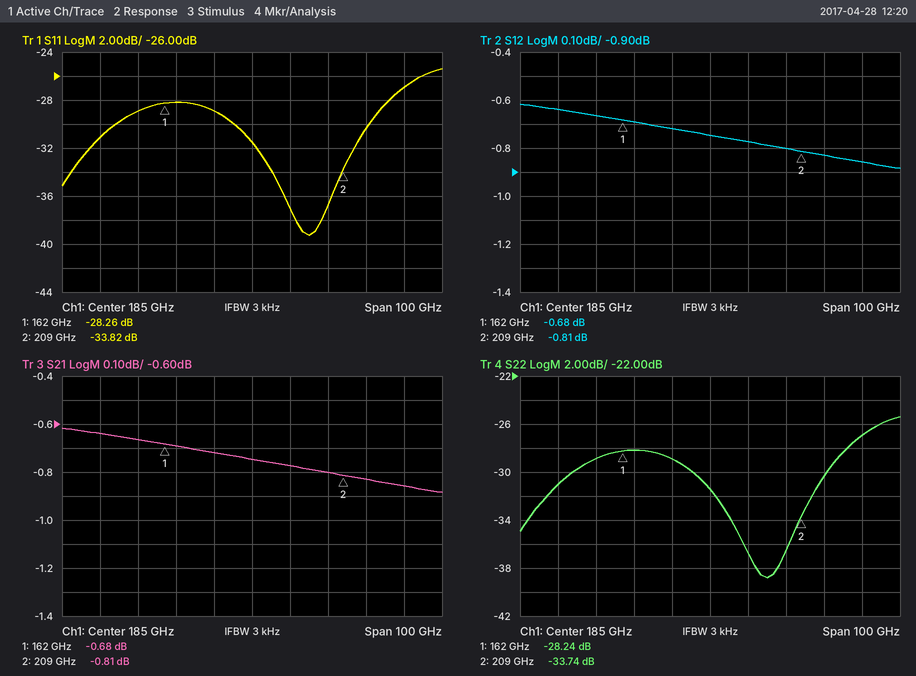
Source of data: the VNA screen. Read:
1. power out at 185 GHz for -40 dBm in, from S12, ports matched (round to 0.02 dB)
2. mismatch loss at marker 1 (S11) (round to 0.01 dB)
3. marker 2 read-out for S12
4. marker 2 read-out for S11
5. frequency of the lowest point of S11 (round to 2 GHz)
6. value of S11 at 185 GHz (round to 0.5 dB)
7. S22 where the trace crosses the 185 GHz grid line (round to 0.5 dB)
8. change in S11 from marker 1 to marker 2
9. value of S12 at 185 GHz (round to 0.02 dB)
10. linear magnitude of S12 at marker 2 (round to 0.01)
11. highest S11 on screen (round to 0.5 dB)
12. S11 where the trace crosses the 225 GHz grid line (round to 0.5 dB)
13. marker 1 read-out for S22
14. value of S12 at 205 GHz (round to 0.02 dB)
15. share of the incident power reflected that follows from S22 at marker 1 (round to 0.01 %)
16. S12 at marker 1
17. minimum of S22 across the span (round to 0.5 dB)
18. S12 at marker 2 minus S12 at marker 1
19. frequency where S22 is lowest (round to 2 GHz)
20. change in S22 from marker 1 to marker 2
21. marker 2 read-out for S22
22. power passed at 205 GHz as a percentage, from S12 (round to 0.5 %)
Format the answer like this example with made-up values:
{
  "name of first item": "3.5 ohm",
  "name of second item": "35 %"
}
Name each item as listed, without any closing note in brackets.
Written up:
{
  "power out at 185 GHz for -40 dBm in, from S12, ports matched": "-40.74 dBm",
  "mismatch loss at marker 1 (S11)": "0.01 dB",
  "marker 2 read-out for S12": "-0.81 dB",
  "marker 2 read-out for S11": "-33.82 dB",
  "frequency of the lowest point of S11": "200 GHz",
  "value of S11 at 185 GHz": "-31.5 dB",
  "S22 where the trace crosses the 185 GHz grid line": "-31.5 dB",
  "change in S11 from marker 1 to marker 2": "-5.56 dB",
  "value of S12 at 185 GHz": "-0.74 dB",
  "linear magnitude of S12 at marker 2": "0.91",
  "highest S11 on screen": "-25.5 dB",
  "S11 where the trace crosses the 225 GHz grid line": "-27.0 dB",
  "marker 1 read-out for S22": "-28.24 dB",
  "value of S12 at 205 GHz": "-0.80 dB",
  "share of the incident power reflected that follows from S22 at marker 1": "0.15 %",
  "S12 at marker 1": "-0.68 dB",
  "minimum of S22 across the span": "-39.0 dB",
  "S12 at marker 2 minus S12 at marker 1": "-0.13 dB",
  "frequency where S22 is lowest": "200 GHz",
  "change in S22 from marker 1 to marker 2": "-5.50 dB",
  "marker 2 read-out for S22": "-33.74 dB",
  "power passed at 205 GHz as a percentage, from S12": "83.0 %"
}
